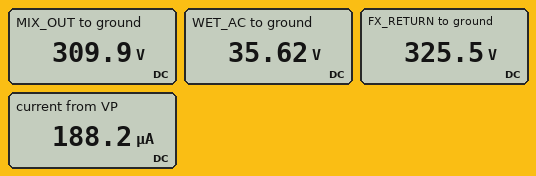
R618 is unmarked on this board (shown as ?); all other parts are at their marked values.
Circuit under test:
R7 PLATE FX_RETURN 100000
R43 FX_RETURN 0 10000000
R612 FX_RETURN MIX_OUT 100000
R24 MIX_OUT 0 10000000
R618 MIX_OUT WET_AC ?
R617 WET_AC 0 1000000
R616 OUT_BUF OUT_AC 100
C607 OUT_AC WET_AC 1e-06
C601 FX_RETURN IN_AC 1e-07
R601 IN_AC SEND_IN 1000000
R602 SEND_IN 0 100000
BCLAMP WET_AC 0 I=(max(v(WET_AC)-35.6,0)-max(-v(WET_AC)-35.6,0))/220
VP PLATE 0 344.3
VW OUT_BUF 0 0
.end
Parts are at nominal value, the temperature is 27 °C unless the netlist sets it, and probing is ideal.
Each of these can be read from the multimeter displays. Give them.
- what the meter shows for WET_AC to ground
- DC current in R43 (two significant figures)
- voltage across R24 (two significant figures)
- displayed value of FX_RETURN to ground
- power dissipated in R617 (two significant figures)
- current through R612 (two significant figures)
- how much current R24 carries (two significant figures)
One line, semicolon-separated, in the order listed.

35.62 V; 33 µA; 310 V; 325.5 V; 1.3 mW; 160 µA; 31 µA
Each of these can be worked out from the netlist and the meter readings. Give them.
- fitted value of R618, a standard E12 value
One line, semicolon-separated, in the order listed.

2.2 MΩ
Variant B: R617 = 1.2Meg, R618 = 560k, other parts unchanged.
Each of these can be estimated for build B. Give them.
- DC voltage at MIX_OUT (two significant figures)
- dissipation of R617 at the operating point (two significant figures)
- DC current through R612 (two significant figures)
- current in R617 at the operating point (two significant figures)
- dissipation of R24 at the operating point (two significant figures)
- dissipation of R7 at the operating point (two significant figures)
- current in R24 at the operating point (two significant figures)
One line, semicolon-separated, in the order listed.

260 V; 1.1 mW; 420 µA; 30 µA; 6.6 mW; 20 mW; 26 µA
